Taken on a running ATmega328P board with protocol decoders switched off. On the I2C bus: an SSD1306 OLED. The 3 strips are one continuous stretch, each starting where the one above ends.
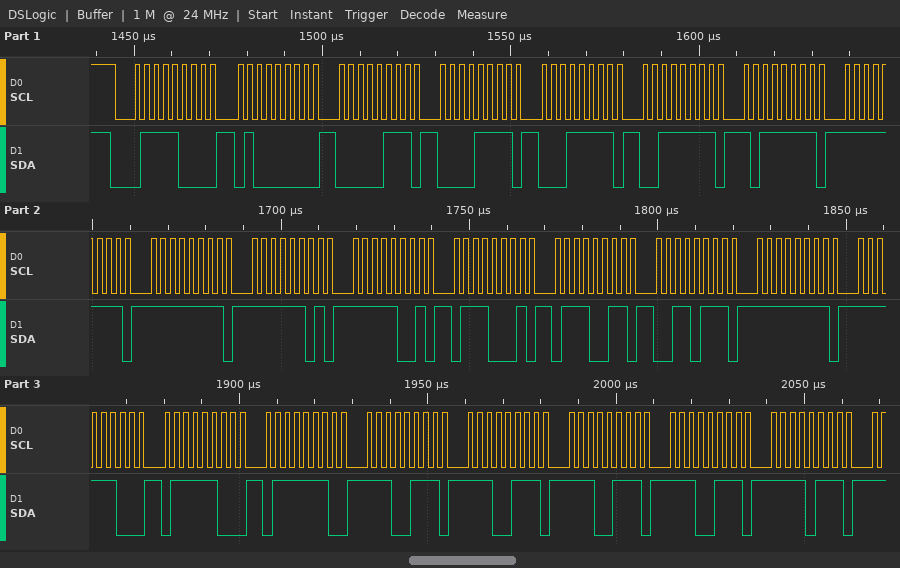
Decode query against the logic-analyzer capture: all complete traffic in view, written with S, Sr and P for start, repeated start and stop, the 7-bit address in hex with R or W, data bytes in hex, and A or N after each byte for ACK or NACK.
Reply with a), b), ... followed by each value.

a) S 3CW A 40 A 07 A 0F A 1F A 3F A BF A FF A FF A FD A F9 A 71 A 73 A 37 A FF A FC A 7C A 7E A E7 A E7 A E7 A E7 A F7 A
